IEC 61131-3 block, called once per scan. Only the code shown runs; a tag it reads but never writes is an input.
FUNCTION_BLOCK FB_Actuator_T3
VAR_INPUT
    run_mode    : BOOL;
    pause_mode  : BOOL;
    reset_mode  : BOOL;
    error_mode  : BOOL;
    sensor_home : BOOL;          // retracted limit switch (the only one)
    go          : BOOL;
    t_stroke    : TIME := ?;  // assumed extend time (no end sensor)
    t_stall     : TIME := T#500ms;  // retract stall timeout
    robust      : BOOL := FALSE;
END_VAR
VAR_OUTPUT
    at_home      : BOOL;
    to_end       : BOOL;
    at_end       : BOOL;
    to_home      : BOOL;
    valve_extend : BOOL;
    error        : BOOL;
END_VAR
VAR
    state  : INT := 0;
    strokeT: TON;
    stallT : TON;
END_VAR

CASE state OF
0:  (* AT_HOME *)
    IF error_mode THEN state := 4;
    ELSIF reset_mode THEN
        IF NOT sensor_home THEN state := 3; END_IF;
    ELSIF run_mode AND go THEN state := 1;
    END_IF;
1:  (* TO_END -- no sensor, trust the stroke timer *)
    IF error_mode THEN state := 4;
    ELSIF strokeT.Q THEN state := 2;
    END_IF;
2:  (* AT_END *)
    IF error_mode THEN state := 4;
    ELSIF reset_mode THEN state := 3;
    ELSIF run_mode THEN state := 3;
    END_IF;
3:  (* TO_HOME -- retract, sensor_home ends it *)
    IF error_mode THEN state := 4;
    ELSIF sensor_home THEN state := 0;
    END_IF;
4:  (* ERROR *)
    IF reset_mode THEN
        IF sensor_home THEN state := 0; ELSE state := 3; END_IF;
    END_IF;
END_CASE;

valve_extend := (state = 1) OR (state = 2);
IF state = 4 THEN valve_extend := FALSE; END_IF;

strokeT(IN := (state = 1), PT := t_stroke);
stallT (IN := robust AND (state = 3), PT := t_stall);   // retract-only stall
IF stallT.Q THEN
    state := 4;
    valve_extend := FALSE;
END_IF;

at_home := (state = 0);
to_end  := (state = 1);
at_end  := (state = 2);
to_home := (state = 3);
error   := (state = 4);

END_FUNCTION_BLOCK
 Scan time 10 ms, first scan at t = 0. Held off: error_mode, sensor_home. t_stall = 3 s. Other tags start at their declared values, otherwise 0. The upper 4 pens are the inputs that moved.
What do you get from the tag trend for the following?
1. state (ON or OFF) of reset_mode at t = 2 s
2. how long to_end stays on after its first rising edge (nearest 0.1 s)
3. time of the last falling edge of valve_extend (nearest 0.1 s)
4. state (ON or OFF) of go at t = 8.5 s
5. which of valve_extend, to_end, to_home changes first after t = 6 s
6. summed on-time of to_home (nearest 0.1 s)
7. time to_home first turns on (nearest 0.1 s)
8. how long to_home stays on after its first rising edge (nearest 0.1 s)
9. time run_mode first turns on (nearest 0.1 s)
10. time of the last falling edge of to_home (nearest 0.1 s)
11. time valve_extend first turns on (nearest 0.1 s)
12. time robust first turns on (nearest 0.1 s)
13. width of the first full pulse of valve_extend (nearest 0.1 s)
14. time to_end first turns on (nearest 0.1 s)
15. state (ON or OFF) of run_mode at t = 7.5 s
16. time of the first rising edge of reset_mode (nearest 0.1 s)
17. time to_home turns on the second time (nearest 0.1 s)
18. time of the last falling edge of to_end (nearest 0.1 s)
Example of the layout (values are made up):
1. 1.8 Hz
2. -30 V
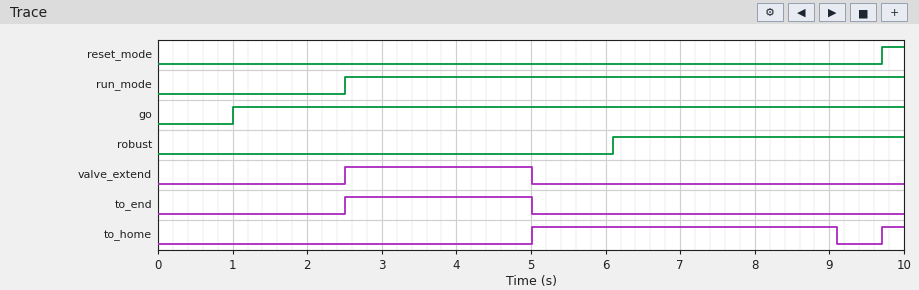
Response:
1. OFF
2. 2.5 s
3. 5.0 s
4. ON
5. to_home
6. 4.4 s
7. 5.0 s
8. 4.1 s
9. 2.5 s
10. 9.1 s
11. 2.5 s
12. 6.1 s
13. 2.5 s
14. 2.5 s
15. ON
16. 9.7 s
17. 9.7 s
18. 5.0 s
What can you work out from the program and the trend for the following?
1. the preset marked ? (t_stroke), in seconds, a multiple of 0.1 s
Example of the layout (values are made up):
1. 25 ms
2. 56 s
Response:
1. 2.5 s
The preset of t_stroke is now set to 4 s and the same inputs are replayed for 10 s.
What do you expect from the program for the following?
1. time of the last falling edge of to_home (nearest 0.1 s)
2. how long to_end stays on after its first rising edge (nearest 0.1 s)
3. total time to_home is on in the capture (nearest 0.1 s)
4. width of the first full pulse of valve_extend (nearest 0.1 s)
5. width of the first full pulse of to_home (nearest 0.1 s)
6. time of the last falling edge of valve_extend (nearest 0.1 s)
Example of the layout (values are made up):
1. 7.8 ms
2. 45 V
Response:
1. 9.5 s
2. 4.0 s
3. 3.3 s
4. 4.0 s
5. 3.0 s
6. 6.5 s
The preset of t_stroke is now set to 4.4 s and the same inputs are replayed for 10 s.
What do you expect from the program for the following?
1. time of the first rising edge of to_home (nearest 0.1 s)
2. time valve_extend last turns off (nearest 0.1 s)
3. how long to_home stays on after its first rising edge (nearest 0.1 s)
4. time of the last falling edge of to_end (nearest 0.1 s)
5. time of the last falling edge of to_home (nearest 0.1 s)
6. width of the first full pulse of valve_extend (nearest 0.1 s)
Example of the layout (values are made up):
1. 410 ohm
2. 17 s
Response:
1. 6.9 s
2. 6.9 s
3. 3.0 s
4. 6.9 s
5. 9.9 s
6. 4.4 s
